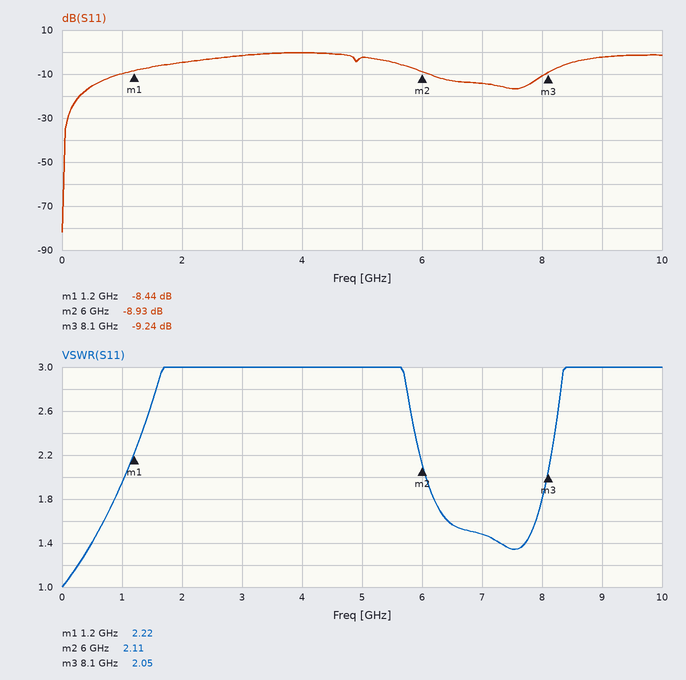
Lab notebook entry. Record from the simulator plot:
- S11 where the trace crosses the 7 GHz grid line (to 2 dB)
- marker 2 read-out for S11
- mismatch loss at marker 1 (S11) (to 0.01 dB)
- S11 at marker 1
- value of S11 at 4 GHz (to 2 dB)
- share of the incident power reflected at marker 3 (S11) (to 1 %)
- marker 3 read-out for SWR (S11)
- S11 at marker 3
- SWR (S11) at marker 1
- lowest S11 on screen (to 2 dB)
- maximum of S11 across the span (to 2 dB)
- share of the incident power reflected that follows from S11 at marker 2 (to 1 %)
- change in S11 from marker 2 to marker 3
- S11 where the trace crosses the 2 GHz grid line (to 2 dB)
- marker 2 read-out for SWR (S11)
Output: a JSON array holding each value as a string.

["-14 dB", "-8.93 dB", "0.67 dB", "-8.44 dB", "0 dB", "12 %", "2.05", "-9.24 dB", "2.22", "-82 dB", "0 dB", "13 %", "-0.31 dB", "-4 dB", "2.11"]
